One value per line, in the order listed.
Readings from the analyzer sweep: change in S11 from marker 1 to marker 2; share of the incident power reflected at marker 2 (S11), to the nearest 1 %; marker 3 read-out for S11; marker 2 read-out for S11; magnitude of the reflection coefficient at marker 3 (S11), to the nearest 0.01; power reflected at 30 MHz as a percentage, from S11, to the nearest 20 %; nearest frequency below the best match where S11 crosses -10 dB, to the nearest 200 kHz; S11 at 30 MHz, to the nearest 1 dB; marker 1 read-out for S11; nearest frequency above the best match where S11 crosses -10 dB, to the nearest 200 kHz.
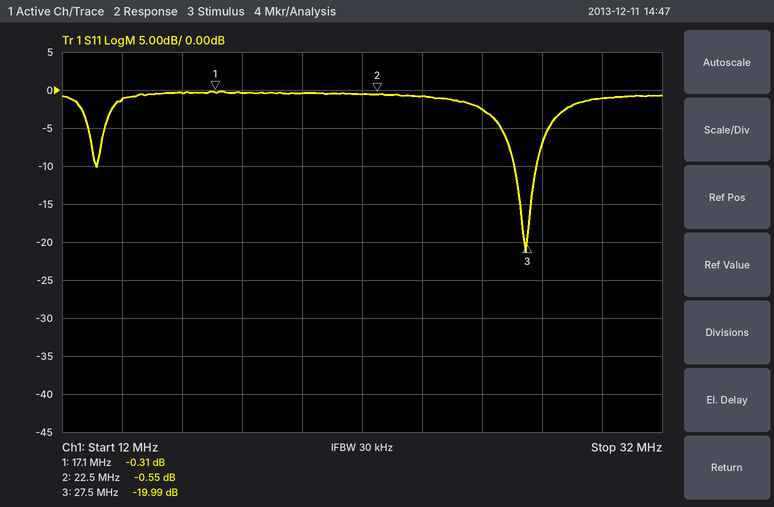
-0.24 dB
88 %
-19.99 dB
-0.55 dB
0.10
80 %
27.0 MHz
-1 dB
-0.31 dB
27.8 MHz
